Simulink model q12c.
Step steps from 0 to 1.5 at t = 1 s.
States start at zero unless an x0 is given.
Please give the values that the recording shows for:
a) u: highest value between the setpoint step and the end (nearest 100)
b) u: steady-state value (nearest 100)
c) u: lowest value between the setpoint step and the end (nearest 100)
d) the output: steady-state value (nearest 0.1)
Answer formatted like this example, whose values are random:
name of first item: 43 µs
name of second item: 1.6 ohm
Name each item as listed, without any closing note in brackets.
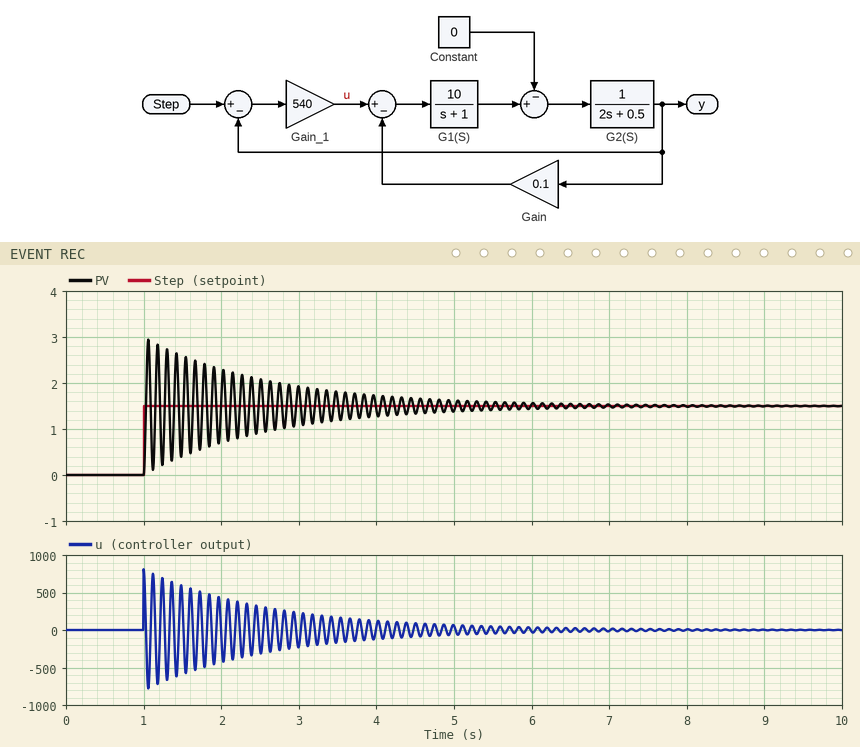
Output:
u: highest value between the setpoint step and the end: 800
u: steady-state value: 0
u: lowest value between the setpoint step and the end: -800
the output: steady-state value: 1.5
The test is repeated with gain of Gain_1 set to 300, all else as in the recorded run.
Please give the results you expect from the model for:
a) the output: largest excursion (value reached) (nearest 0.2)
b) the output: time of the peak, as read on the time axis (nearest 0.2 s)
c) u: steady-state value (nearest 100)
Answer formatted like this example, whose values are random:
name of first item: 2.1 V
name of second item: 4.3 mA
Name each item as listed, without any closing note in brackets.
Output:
the output: largest excursion (value reached): 3.0
the output: time of the peak, as read on the time axis: 1.0 s
u: steady-state value: 0
